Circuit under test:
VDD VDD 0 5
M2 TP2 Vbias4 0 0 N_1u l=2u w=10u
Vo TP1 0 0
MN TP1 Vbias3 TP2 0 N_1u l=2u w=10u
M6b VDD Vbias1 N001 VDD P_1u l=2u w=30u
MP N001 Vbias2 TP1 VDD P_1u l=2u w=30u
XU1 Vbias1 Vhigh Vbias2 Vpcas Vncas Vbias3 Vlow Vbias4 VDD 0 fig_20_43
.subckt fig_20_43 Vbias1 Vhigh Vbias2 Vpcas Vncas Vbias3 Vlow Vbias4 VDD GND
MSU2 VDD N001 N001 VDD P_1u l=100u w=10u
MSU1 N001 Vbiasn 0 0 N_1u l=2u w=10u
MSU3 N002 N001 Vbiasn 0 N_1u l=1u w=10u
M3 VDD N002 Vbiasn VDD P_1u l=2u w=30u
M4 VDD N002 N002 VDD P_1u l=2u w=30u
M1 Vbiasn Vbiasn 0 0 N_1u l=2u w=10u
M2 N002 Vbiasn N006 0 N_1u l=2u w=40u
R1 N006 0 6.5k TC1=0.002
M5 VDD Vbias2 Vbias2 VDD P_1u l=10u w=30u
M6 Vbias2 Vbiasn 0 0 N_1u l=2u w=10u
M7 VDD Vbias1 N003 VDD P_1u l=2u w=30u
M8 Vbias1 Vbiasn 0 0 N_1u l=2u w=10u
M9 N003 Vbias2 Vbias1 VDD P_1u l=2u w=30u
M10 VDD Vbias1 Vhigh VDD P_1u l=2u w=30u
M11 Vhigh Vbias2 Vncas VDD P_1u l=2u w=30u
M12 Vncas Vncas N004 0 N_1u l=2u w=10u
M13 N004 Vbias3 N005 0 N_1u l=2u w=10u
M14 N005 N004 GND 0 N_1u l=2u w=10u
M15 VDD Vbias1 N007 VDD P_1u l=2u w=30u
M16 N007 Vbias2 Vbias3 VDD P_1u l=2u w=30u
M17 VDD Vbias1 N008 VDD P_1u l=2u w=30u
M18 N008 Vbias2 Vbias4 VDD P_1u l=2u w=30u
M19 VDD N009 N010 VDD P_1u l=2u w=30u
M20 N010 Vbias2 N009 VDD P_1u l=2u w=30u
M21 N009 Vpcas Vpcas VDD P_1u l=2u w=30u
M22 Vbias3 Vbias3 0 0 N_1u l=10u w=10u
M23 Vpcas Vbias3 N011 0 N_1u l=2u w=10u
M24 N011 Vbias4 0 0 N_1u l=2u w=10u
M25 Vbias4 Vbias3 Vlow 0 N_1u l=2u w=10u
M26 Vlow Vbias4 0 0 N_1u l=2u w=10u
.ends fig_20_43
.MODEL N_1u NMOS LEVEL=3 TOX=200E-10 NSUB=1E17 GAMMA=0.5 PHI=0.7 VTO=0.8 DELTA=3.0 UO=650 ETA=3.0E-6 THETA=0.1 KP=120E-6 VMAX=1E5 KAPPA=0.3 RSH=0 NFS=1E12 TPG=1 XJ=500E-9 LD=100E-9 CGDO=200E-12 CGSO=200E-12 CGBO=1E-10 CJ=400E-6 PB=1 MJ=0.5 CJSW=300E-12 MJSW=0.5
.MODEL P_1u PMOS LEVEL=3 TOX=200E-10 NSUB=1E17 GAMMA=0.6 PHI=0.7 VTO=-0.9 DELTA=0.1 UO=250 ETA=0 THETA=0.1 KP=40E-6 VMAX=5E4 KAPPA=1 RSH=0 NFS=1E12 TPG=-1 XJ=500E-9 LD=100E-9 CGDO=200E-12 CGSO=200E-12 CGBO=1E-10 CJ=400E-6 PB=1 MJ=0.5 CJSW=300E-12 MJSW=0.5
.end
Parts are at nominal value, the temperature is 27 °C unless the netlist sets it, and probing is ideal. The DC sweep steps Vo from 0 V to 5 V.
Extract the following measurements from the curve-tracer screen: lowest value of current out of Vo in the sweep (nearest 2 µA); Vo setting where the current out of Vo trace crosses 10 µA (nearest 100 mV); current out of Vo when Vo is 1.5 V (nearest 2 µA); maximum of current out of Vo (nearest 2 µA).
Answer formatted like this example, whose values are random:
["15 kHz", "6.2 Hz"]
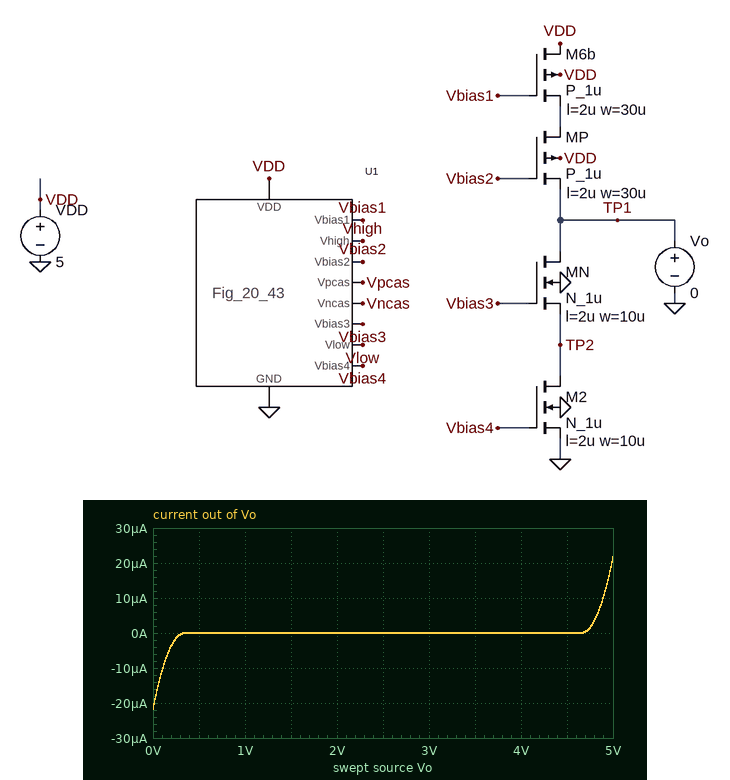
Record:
["-22 µA", "4.9 V", "0 A", "22 µA"]
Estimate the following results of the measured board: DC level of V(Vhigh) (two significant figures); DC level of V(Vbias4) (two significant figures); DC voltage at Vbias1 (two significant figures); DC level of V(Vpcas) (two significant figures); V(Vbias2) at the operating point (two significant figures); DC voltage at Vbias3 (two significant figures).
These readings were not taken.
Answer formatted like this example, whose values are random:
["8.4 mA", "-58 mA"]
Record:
["4.7 V", "1.1 V", "3.8 V", "2.4 V", "3.4 V", "1.5 V"]
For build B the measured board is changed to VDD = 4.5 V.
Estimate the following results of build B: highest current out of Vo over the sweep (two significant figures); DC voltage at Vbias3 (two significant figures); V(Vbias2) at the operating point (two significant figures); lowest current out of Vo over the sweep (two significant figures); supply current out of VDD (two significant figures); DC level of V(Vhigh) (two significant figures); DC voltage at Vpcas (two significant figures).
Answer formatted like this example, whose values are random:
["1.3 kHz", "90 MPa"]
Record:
["130 µA", "1.5 V", "2.9 V", "-21 µA", "200 µA", "4.2 V", "1.9 V"]
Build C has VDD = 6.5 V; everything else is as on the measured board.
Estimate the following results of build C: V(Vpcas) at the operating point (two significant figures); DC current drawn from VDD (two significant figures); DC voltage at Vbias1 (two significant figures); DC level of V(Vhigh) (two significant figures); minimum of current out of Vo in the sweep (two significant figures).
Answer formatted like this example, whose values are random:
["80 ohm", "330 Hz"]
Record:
["3.9 V", "230 µA", "5.3 V", "6.2 V", "-23 µA"]
